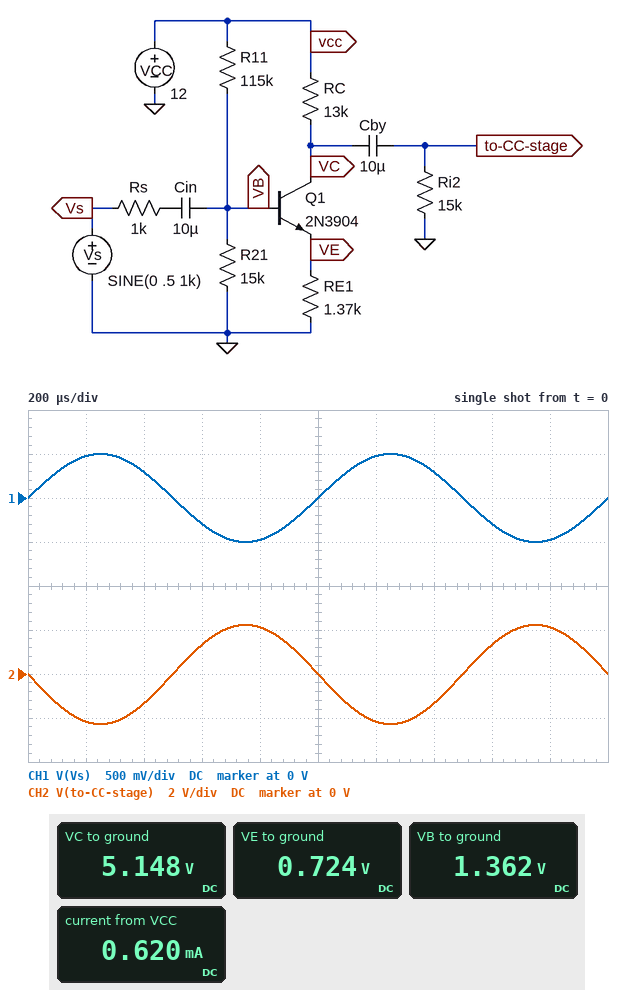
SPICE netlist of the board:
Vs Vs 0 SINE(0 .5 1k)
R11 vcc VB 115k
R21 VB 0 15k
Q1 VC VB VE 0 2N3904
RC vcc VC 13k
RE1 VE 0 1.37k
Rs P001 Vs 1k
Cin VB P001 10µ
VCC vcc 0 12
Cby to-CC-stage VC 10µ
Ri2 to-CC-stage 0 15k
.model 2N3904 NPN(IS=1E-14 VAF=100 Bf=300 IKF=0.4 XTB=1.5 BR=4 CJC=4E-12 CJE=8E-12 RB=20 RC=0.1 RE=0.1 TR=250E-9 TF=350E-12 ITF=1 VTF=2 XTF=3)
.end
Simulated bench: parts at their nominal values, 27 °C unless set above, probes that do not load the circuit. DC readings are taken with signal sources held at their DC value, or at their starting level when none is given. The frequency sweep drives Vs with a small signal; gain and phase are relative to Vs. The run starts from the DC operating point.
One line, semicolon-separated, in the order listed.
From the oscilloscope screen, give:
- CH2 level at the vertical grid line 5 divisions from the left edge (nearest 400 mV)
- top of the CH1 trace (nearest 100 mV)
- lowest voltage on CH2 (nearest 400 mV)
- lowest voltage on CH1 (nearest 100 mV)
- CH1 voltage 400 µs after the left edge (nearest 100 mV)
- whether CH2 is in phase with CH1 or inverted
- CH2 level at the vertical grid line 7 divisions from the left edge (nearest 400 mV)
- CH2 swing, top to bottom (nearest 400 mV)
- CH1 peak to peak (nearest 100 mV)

0 V; 500 mV; -2.4 V; -500 mV; 300 mV; inverted; -1.2 V; 4.4 V; 1.0 V
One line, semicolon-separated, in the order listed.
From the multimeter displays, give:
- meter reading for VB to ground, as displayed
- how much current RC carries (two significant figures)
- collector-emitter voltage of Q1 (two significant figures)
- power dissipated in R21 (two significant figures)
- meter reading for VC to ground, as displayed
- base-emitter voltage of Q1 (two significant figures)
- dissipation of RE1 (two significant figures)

1.362 V; 530 µA; 4.4 V; 120 µW; 5.148 V; 640 mV; 380 µW
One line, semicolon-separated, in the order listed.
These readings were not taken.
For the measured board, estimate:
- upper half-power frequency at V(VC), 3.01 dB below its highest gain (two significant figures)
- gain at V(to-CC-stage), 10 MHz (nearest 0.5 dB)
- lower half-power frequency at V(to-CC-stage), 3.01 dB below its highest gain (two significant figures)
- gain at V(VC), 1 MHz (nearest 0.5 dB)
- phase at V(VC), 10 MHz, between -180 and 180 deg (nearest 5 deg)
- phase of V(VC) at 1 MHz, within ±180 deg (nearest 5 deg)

5.7 MHz; 7.0 dB; 1.4 Hz; 13.0 dB; 105 deg; 170 deg
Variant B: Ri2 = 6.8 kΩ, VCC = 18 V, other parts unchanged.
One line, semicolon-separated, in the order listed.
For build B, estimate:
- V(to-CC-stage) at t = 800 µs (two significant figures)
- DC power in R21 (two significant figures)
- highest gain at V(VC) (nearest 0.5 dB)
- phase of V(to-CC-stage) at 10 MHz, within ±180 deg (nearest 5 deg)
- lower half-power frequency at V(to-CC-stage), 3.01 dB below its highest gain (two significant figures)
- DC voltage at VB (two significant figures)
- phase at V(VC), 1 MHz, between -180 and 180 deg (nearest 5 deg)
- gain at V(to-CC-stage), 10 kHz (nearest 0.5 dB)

1.4 V; 280 µW; 12.0 dB; 115 deg; 1.5 Hz; 2.0 V; 170 deg; 9.5 dB
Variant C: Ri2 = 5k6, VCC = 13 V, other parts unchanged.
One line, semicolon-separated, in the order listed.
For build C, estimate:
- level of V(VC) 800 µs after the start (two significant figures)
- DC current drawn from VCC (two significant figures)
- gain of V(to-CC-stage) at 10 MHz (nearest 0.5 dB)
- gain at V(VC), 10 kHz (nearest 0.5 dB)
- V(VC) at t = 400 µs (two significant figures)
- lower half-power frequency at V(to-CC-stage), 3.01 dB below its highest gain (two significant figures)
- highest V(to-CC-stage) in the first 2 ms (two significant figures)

6.3 V; 710 µA; 5.0 dB; 8.0 dB; 4.4 V; 1.6 Hz; 1.3 V
